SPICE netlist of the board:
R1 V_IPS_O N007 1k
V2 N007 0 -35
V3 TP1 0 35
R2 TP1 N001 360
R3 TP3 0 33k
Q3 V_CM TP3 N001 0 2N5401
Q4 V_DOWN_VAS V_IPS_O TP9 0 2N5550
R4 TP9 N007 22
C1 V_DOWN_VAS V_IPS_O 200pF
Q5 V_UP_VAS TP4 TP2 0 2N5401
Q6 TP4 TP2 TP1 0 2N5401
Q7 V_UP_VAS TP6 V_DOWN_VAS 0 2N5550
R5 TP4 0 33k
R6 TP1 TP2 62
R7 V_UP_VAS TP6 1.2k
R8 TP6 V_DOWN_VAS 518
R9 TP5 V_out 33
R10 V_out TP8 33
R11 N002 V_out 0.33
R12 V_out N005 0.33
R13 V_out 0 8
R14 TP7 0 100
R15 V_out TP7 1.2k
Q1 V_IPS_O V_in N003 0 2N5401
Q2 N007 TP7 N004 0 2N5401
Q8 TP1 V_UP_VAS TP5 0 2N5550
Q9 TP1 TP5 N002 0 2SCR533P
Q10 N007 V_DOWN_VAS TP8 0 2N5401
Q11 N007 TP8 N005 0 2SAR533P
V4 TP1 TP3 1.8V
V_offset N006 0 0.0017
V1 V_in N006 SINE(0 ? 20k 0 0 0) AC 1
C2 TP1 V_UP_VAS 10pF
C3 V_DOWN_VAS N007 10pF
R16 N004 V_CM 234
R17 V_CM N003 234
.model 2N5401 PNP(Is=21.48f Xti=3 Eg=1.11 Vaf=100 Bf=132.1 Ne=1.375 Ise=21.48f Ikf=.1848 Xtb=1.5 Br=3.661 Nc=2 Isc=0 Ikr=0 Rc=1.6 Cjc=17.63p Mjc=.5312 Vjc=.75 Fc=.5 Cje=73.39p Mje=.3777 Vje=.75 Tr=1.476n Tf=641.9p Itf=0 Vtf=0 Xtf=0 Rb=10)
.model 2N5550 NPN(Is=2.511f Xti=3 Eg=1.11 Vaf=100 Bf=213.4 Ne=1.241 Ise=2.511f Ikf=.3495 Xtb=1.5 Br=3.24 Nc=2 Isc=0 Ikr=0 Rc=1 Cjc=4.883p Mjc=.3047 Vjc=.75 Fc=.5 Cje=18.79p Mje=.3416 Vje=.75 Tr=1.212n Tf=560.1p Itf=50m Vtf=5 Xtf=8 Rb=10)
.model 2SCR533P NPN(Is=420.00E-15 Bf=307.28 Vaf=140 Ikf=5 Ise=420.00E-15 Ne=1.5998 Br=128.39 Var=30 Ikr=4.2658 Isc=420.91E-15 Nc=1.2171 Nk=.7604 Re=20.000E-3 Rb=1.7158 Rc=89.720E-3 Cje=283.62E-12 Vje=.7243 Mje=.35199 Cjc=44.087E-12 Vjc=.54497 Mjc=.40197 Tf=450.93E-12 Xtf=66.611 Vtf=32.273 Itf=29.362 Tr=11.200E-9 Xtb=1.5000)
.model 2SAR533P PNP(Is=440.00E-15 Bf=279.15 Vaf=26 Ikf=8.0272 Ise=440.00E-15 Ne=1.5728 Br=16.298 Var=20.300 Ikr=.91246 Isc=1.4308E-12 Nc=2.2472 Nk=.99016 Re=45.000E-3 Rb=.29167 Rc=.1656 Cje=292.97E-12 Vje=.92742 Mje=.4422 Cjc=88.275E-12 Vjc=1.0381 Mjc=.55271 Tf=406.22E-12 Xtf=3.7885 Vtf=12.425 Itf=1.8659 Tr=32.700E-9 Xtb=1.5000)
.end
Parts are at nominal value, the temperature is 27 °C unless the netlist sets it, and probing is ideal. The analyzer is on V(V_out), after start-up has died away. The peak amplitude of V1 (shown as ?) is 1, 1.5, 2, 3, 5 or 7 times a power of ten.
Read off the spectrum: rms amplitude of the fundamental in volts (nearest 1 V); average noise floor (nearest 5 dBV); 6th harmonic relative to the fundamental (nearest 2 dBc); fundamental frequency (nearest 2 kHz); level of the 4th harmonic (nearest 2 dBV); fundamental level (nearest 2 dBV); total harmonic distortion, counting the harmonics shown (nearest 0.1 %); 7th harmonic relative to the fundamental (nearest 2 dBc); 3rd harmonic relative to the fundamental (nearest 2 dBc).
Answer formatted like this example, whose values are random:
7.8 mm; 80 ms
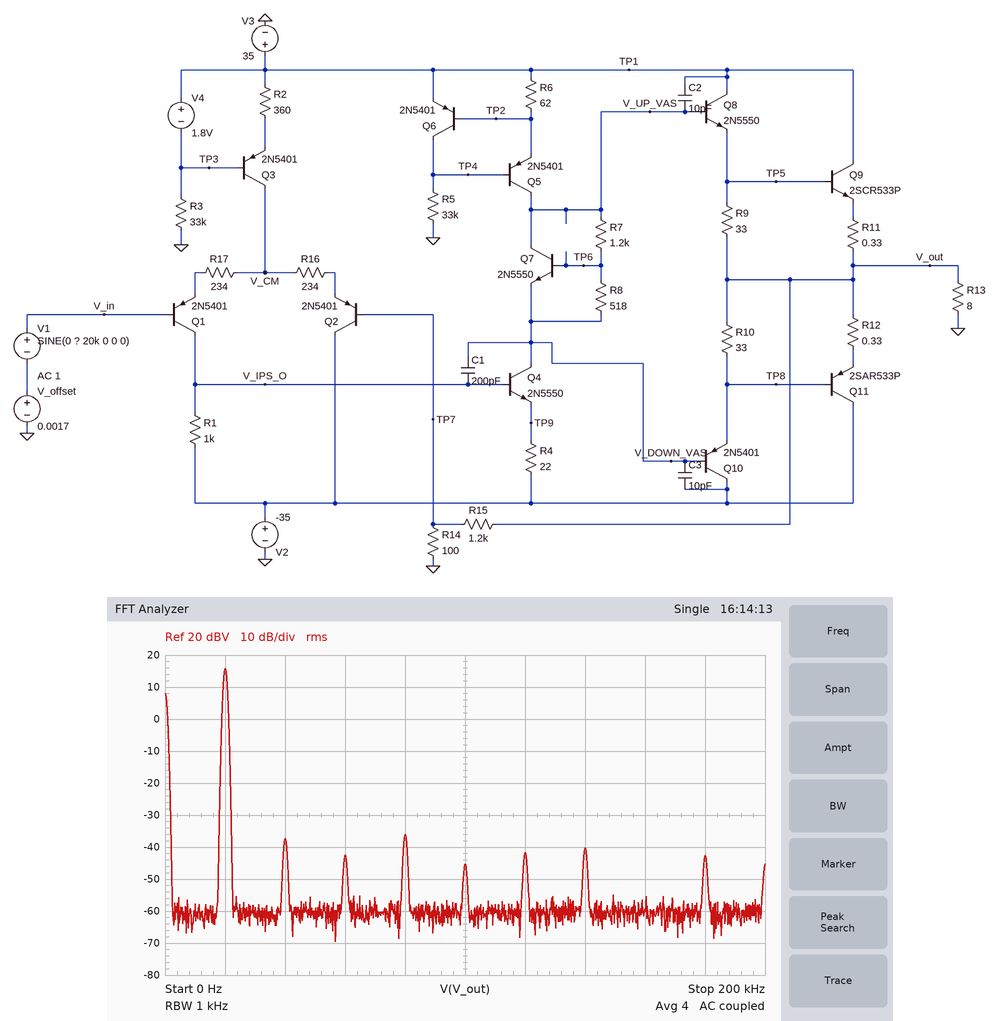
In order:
6 V; -60 dBV; -58 dBc; 20 kHz; -36 dBV; 16 dBV; 0.4 %; -56 dBc; -58 dBc
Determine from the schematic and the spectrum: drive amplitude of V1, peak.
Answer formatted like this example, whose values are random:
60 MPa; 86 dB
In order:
700 mV
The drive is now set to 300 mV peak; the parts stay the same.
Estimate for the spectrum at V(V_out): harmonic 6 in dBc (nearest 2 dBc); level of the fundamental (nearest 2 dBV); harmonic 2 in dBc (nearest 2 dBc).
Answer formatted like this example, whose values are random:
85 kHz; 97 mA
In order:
-60 dBc; 8 dBV; -46 dBc
